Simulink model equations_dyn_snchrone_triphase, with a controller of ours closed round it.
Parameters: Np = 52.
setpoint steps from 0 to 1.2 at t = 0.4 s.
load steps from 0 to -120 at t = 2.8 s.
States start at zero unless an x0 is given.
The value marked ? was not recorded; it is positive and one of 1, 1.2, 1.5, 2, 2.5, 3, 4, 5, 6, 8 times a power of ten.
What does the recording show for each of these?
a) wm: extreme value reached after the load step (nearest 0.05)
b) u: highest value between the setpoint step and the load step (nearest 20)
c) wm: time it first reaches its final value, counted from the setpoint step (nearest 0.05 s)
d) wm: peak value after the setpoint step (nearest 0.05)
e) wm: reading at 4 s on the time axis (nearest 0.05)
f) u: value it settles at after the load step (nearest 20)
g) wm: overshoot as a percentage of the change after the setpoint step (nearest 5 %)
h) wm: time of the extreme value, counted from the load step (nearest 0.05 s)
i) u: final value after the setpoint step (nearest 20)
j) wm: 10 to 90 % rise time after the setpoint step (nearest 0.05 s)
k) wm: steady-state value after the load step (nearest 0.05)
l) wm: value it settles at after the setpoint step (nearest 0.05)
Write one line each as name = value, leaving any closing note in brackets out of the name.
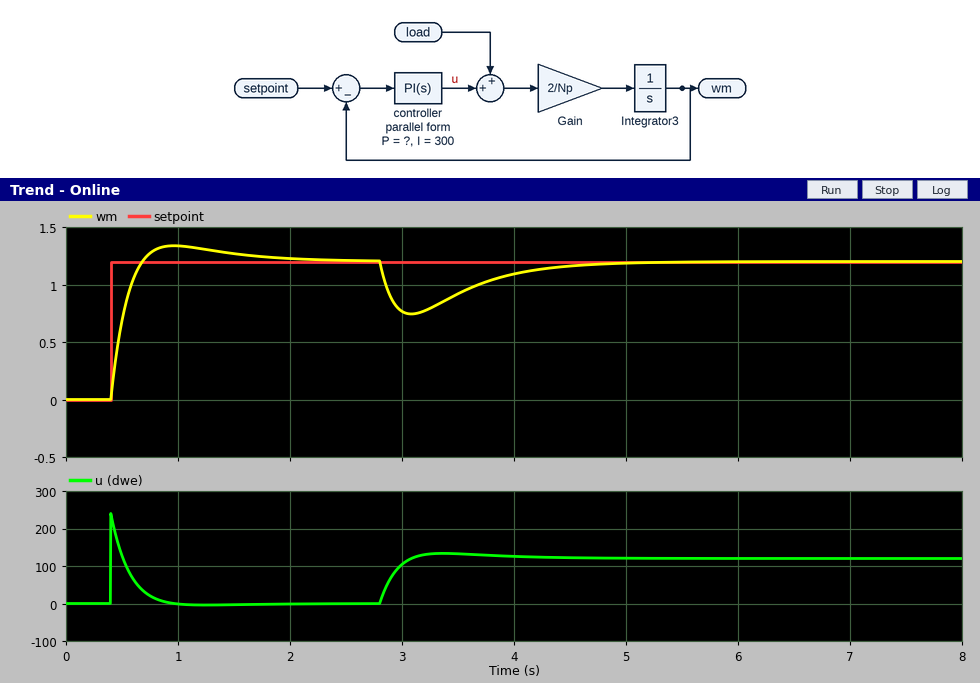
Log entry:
wm: extreme value reached after the load step = 0.75
u: highest value between the setpoint step and the load step = 240
wm: time it first reaches its final value, counted from the setpoint step = 0.30 s
wm: peak value after the setpoint step = 1.35
wm: reading at 4 s on the time axis = 1.10
u: value it settles at after the load step = 120
wm: overshoot as a percentage of the change after the setpoint step = 10 %
wm: time of the extreme value, counted from the load step = 0.30 s
u: final value after the setpoint step = 0
wm: 10 to 90 % rise time after the setpoint step = 0.20 s
wm: steady-state value after the load step = 1.20
wm: value it settles at after the setpoint step = 1.20
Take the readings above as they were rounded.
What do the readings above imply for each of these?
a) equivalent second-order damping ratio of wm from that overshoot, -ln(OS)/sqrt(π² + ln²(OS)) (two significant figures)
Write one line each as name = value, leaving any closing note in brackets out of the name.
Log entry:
equivalent second-order damping ratio of wm from that overshoot, -ln(OS)/sqrt(π² + ln²(OS)) = 0.59
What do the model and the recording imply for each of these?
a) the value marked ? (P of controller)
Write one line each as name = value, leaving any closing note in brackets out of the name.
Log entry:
the value marked ? = 200
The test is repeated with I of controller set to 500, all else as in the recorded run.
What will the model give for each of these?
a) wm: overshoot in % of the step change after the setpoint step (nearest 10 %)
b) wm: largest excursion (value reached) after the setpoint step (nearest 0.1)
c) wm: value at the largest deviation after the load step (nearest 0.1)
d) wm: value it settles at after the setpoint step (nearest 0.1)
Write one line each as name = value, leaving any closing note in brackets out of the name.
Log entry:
wm: overshoot in % of the step change after the setpoint step = 20 %
wm: largest excursion (value reached) after the setpoint step = 1.4
wm: value at the largest deviation after the load step = 0.8
wm: value it settles at after the setpoint step = 1.2
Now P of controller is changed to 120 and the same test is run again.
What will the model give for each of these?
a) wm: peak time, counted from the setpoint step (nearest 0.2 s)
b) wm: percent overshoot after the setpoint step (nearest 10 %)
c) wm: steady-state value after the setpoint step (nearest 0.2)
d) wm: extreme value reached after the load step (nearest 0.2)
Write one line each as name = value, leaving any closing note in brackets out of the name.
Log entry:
wm: peak time, counted from the setpoint step = 0.6 s
wm: percent overshoot after the setpoint step = 20 %
wm: steady-state value after the setpoint step = 1.2
wm: extreme value reached after the load step = 0.6
